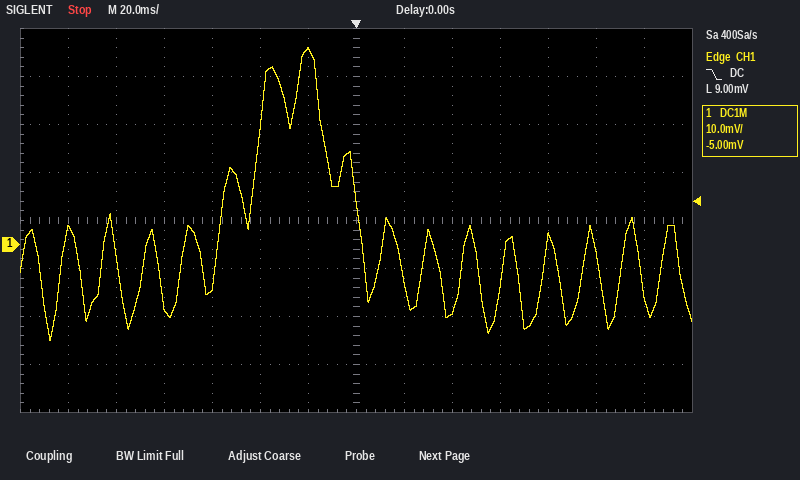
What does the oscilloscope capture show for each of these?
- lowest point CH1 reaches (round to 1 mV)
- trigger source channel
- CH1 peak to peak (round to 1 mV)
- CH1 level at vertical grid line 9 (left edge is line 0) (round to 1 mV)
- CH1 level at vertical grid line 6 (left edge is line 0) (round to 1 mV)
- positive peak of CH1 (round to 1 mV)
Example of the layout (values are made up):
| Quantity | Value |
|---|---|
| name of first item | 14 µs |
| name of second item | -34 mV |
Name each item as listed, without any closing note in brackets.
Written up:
| Quantity | Value |
|---|---|
| lowest point CH1 reaches | -20 mV |
| trigger source channel | CH1 |
| CH1 peak to peak | 61 mV |
| CH1 level at vertical grid line 9 (left edge is line 0) | -14 mV |
| CH1 level at vertical grid line 6 (left edge is line 0) | 41 mV |
| positive peak of CH1 | 41 mV |
